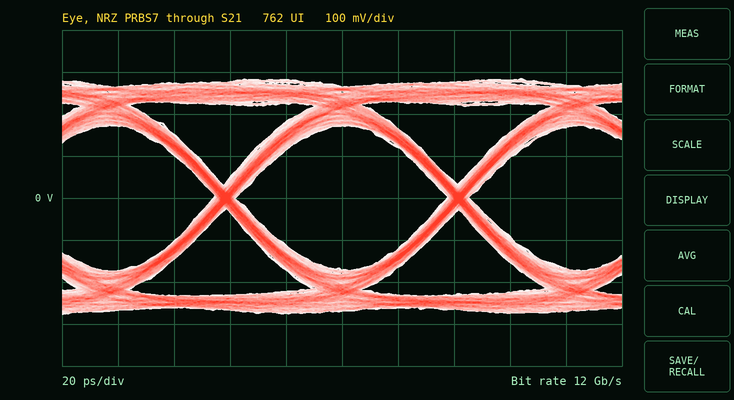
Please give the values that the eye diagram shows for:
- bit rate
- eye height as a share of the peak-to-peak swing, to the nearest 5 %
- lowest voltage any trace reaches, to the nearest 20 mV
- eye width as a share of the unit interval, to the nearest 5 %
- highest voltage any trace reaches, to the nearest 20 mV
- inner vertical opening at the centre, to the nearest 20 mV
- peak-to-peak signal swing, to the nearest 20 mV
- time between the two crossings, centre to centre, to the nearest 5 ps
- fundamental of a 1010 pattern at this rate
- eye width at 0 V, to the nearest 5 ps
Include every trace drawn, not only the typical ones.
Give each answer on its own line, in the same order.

12 Gb/s
60 %
-280 mV
90 %
280 mV
340 mV
560 mV
85 ps
6 GHz
75 ps
